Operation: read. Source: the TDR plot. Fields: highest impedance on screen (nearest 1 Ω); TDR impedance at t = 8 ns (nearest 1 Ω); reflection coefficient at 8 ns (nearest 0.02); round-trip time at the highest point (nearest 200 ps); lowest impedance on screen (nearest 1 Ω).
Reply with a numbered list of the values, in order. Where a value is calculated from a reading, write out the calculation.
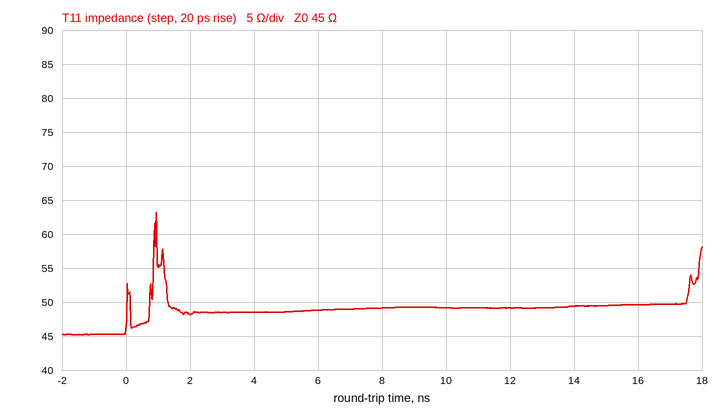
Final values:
1. 63 Ω
2. 49 Ω
3. (49 − 45)/(49 + 45) ≈ +0.04
4. 1.0 ns
5. 45 Ω
